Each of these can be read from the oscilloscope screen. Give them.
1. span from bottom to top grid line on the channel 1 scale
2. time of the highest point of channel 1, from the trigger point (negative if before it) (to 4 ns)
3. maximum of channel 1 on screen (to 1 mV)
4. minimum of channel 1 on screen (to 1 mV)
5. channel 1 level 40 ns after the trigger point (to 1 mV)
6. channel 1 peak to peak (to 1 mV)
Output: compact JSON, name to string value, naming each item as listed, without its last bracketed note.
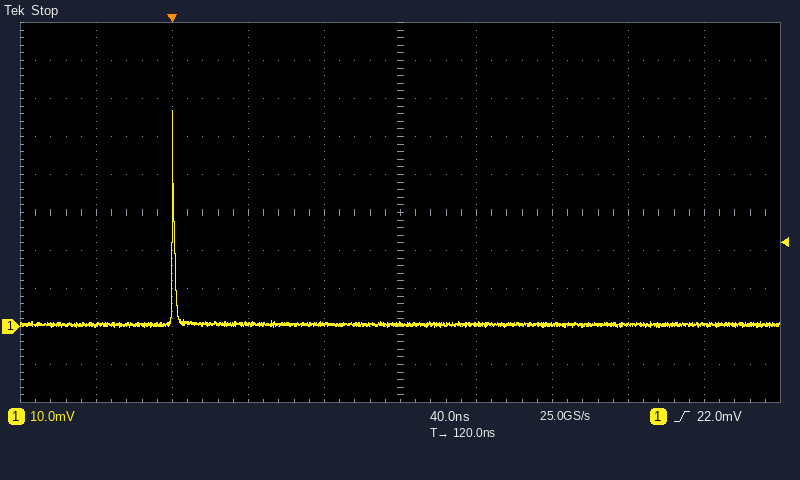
{"span from bottom to top grid line on the channel 1 scale": "100 mV", "time of the highest point of channel 1, from the trigger point (negative if before it)": "0 ns", "maximum of channel 1 on screen": "57 mV", "minimum of channel 1 on screen": "0 mV", "channel 1 level 40 ns after the trigger point": "1 mV", "channel 1 peak to peak": "57 mV"}
